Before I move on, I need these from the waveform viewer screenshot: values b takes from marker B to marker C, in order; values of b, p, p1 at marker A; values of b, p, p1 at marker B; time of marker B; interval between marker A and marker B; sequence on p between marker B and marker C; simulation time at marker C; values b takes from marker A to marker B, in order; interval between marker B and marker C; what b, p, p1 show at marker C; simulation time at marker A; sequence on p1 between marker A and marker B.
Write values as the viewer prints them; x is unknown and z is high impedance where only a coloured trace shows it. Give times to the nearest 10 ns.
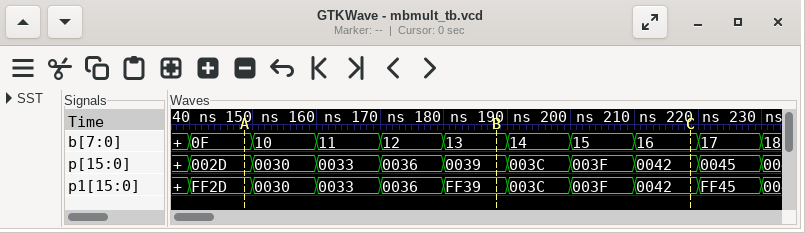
13, 14, 15, 16
b=0F, p=002D, p1=FF2D
b=13, p=0039, p1=FF39
190 ns
40 ns
0039, 003C, 003F, 0042
220 ns
0F, 10, 11, 12, 13
30 ns
b=16, p=0042, p1=0042
150 ns
FF2D, 0030, 0033, 0036, FF39
